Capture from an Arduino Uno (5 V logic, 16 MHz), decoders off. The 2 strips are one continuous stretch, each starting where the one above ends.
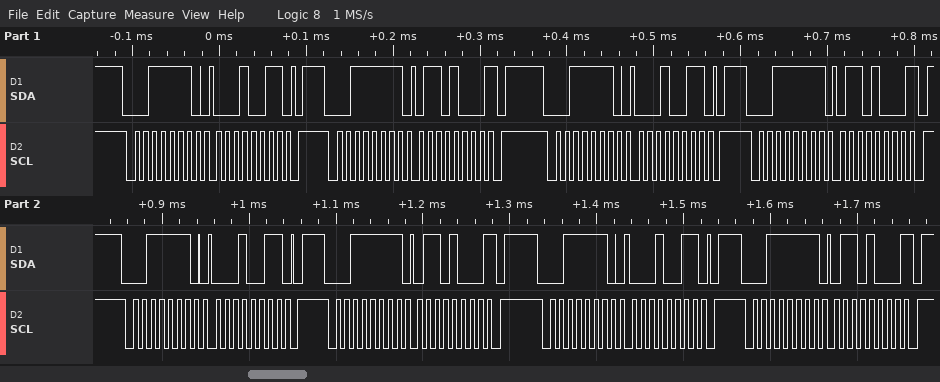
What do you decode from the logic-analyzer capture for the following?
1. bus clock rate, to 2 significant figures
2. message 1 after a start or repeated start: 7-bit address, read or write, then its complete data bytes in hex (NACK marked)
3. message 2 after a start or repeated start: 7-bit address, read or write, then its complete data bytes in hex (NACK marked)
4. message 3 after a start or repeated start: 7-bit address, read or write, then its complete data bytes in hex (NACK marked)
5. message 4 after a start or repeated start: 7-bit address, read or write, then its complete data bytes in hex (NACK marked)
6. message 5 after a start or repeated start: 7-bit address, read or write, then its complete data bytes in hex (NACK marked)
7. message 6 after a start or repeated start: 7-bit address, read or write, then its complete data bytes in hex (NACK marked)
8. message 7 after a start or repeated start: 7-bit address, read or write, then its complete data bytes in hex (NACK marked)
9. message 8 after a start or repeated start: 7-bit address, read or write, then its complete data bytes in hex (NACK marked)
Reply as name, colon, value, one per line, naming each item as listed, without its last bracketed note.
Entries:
bus clock rate, to 2 significant figures: 100 kHz
message 1 after a start or repeated start: 7-bit address, read or write, then its complete data bytes in hex: 0x1F write: 13
message 2 after a start or repeated start: 7-bit address, read or write, then its complete data bytes in hex: 0x1F read: 68 NACK
message 3 after a start or repeated start: 7-bit address, read or write, then its complete data bytes in hex: 0x1F write: 13
message 4 after a start or repeated start: 7-bit address, read or write, then its complete data bytes in hex: 0x1F read: 68 NACK
message 5 after a start or repeated start: 7-bit address, read or write, then its complete data bytes in hex: 0x1F write: 13
message 6 after a start or repeated start: 7-bit address, read or write, then its complete data bytes in hex: 0x1F read: 68 NACK
message 7 after a start or repeated start: 7-bit address, read or write, then its complete data bytes in hex: 0x1F write: 13
message 8 after a start or repeated start: 7-bit address, read or write, then its complete data bytes in hex: 0x1F read: 68 NACK
